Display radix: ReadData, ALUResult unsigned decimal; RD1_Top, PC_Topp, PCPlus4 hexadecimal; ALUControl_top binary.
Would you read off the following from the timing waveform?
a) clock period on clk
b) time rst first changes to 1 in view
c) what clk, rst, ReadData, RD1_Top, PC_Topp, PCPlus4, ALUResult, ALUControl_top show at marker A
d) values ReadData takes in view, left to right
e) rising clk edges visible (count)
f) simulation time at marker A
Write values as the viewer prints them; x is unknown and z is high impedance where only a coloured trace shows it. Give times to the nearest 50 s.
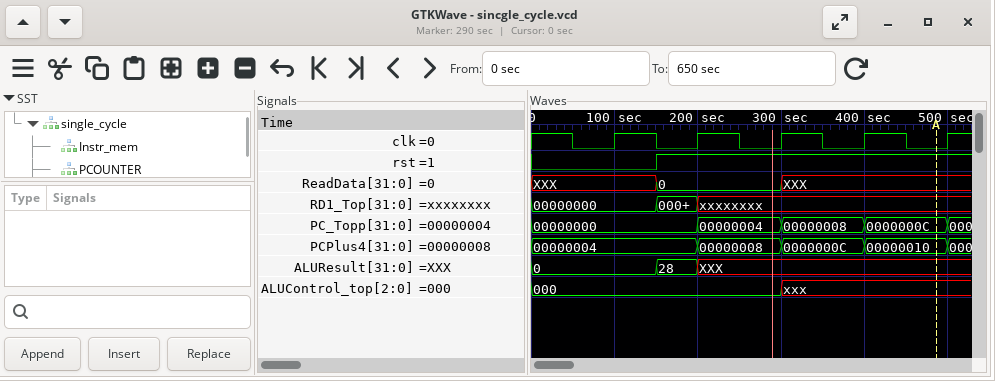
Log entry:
100 s
150 s
clk=0, rst=1, ReadData=XXX, RD1_Top=xxxxxxxx, PC_Topp=0000000C, PCPlus4=00000010, ALUResult=XXX, ALUControl_top=xxx
XXX, 0, XXX
5
500 s
